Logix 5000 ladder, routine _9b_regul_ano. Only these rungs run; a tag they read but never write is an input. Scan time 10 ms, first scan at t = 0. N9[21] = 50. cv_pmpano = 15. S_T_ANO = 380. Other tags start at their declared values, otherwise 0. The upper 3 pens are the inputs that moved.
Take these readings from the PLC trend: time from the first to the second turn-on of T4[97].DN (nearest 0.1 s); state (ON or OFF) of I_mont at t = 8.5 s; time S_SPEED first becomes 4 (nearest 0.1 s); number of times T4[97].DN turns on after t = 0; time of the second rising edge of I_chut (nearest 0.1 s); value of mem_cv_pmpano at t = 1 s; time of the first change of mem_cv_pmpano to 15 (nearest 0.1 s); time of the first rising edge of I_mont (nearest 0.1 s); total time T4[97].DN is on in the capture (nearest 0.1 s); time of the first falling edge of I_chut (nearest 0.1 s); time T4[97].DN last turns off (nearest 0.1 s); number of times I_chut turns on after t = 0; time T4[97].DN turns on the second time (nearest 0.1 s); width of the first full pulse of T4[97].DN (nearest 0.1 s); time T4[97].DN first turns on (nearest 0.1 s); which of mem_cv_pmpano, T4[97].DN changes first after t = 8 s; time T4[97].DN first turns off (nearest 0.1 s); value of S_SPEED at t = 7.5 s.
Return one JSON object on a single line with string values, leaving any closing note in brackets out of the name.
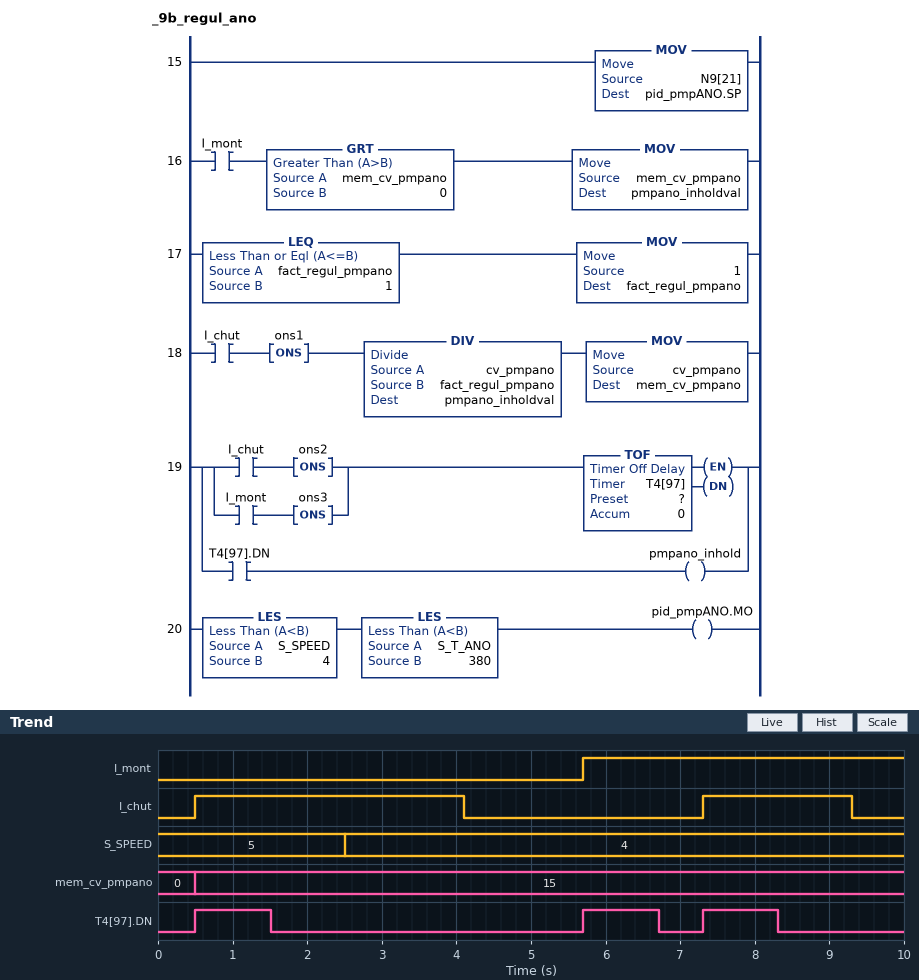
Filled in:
{"time from the first to the second turn-on of T4[97].DN": "5.2 s", "state (ON or OFF) of I_mont at t = 8.5 s": "ON", "time S_SPEED first becomes 4": "2.5 s", "number of times T4[97].DN turns on after t = 0": "3", "time of the second rising edge of I_chut": "7.3 s", "value of mem_cv_pmpano at t = 1 s": "15", "time of the first change of mem_cv_pmpano to 15": "0.5 s", "time of the first rising edge of I_mont": "5.7 s", "total time T4[97].DN is on in the capture": "3.0 s", "time of the first falling edge of I_chut": "4.1 s", "time T4[97].DN last turns off": "8.3 s", "number of times I_chut turns on after t = 0": "2", "time T4[97].DN turns on the second time": "5.7 s", "width of the first full pulse of T4[97].DN": "1.0 s", "time T4[97].DN first turns on": "0.5 s", "which of mem_cv_pmpano, T4[97].DN changes first after t = 8 s": "T4[97].DN", "time T4[97].DN first turns off": "1.5 s", "value of S_SPEED at t = 7.5 s": "4"}
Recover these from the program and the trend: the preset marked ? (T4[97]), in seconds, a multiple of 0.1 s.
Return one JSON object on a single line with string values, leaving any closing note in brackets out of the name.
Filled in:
{"the preset marked ? (T4[97]), in seconds, a multiple of 0.1 s": "1.0 s"}
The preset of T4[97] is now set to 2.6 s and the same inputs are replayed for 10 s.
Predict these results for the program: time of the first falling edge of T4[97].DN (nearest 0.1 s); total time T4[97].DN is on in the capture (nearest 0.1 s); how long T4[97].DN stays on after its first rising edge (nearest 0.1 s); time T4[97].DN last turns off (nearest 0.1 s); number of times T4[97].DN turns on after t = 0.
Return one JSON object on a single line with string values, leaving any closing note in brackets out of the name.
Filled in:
{"time of the first falling edge of T4[97].DN": "3.1 s", "total time T4[97].DN is on in the capture": "6.8 s", "how long T4[97].DN stays on after its first rising edge": "2.6 s", "time T4[97].DN last turns off": "9.9 s", "number of times T4[97].DN turns on after t = 0": "2"}
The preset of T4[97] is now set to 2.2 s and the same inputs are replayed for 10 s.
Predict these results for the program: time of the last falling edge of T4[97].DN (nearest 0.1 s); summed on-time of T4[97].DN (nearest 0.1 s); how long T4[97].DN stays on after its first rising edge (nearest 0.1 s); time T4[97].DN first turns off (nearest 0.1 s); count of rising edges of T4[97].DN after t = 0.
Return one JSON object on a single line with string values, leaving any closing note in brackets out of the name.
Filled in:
{"time of the last falling edge of T4[97].DN": "9.5 s", "summed on-time of T4[97].DN": "6.0 s", "how long T4[97].DN stays on after its first rising edge": "2.2 s", "time T4[97].DN first turns off": "2.7 s", "count of rising edges of T4[97].DN after t = 0": "2"}
